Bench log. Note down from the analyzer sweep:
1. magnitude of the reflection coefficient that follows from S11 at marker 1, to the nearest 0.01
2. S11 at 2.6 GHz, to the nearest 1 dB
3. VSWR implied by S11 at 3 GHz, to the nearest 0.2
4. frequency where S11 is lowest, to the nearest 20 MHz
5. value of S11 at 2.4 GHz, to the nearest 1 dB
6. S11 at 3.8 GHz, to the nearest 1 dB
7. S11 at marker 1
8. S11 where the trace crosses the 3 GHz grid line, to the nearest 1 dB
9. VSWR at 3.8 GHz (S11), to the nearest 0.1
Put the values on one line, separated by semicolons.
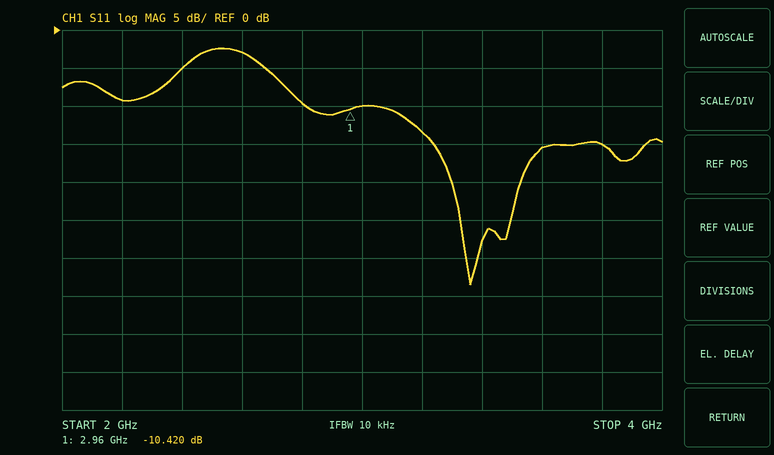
0.30; -3 dB; 2.0; 3.36 GHz; -5 dB; -15 dB; -10.420 dB; -10 dB; 1.4
